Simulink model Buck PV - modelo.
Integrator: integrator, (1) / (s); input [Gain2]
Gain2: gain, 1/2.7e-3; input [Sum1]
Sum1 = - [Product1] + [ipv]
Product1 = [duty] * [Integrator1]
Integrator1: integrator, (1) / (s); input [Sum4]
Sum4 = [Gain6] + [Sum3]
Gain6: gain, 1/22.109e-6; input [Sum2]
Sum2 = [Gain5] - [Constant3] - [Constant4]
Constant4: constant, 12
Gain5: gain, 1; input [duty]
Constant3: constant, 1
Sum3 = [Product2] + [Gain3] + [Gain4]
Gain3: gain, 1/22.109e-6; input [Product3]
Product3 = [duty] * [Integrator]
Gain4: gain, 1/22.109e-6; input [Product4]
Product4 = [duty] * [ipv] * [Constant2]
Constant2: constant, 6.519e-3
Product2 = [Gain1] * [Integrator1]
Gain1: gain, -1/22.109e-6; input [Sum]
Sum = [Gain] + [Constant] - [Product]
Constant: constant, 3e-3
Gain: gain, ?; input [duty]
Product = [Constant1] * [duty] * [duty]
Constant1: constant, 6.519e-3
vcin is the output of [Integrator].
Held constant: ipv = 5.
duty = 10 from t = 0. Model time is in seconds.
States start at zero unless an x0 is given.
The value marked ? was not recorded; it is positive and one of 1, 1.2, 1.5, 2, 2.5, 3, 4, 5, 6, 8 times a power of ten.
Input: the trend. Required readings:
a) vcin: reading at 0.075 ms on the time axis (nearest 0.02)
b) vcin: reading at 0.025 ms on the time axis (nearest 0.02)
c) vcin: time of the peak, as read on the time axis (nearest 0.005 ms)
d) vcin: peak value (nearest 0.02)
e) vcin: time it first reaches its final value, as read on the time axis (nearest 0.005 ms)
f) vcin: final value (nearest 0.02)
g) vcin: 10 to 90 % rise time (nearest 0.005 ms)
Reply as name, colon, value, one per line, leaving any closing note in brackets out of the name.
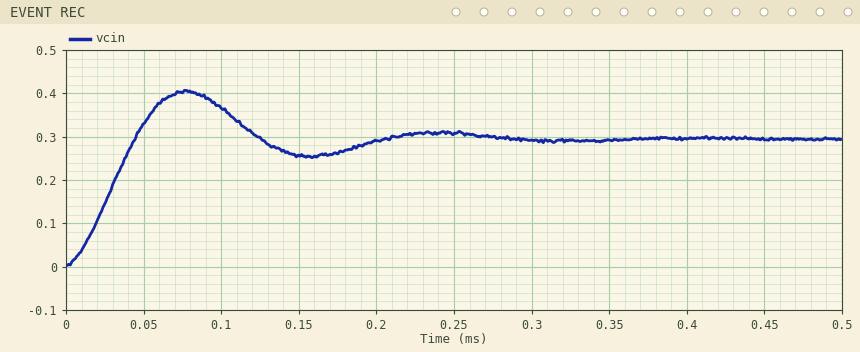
vcin: reading at 0.075 ms on the time axis: 0.40
vcin: reading at 0.025 ms on the time axis: 0.14
vcin: time of the peak, as read on the time axis: 0.075 ms
vcin: peak value: 0.40
vcin: time it first reaches its final value, as read on the time axis: 0.045 ms
vcin: final value: 0.30
vcin: 10 to 90 % rise time: 0.030 ms
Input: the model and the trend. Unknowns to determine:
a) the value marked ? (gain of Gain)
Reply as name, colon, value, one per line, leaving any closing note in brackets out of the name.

the value marked ?: 0.12
